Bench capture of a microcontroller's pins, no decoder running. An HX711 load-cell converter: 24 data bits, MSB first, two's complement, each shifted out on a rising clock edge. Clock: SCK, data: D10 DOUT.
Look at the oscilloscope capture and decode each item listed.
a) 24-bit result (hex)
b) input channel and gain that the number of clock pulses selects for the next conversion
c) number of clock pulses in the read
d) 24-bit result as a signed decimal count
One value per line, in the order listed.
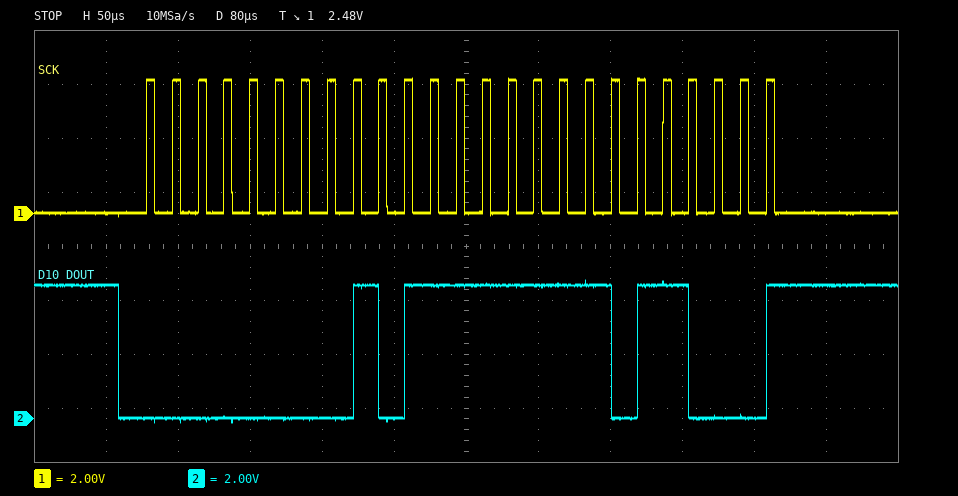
0x00BFD8
channel A, gain 128
25
49112
